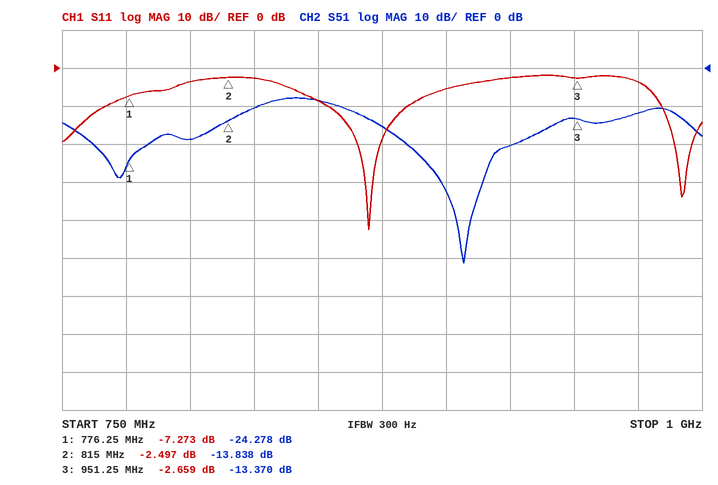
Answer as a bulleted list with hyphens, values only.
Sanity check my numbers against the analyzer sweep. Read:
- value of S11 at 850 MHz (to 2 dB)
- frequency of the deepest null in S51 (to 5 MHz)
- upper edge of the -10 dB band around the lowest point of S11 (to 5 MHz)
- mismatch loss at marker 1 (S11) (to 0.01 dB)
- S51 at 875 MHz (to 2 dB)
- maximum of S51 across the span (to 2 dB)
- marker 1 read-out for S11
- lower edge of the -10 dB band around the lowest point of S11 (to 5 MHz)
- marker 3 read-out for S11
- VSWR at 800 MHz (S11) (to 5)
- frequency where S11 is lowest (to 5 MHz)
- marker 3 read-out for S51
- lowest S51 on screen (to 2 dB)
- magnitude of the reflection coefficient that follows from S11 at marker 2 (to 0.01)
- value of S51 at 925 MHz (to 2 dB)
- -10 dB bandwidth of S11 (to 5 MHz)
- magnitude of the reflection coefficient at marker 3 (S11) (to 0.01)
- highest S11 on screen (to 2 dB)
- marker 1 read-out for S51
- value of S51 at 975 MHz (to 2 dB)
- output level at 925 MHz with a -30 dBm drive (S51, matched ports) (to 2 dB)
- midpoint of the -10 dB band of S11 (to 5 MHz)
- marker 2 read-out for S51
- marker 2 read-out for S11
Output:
- -8 dB
- 905 MHz
- 885 MHz
- 0.90 dB
- -16 dB
- -8 dB
- -7.273 dB
- 855 MHz
- -2.659 dB
- 5
- 870 MHz
- -13.370 dB
- -52 dB
- 0.75
- -20 dB
- 30 MHz
- 0.74
- -2 dB
- -24.278 dB
- -12 dB
- -50 dBm
- 870 MHz
- -13.838 dB
- -2.497 dB
